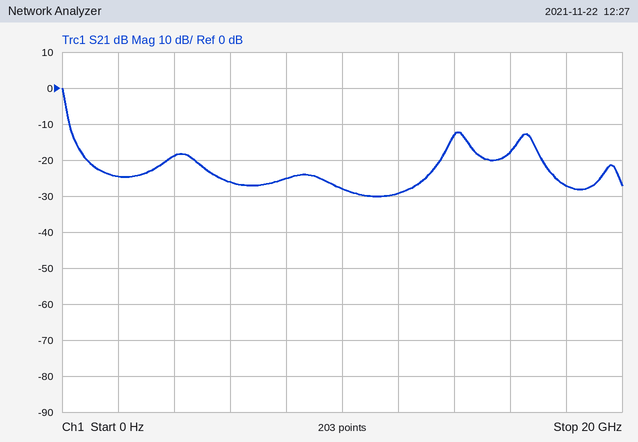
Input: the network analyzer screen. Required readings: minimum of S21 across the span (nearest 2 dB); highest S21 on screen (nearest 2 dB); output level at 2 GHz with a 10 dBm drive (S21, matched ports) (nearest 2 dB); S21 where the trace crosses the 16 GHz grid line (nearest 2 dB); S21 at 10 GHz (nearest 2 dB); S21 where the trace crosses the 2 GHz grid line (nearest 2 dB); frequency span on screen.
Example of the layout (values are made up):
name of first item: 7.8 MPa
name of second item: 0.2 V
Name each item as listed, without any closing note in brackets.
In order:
minimum of S21 across the span: -30 dB
highest S21 on screen: 0 dB
output level at 2 GHz with a 10 dBm drive (S21, matched ports): -14 dBm
S21 where the trace crosses the 16 GHz grid line: -18 dB
S21 at 10 GHz: -28 dB
S21 where the trace crosses the 2 GHz grid line: -24 dB
frequency span on screen: 20 GHz
